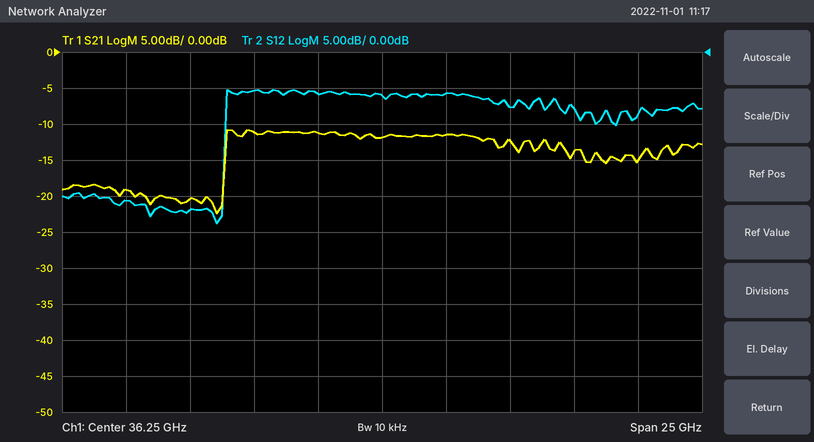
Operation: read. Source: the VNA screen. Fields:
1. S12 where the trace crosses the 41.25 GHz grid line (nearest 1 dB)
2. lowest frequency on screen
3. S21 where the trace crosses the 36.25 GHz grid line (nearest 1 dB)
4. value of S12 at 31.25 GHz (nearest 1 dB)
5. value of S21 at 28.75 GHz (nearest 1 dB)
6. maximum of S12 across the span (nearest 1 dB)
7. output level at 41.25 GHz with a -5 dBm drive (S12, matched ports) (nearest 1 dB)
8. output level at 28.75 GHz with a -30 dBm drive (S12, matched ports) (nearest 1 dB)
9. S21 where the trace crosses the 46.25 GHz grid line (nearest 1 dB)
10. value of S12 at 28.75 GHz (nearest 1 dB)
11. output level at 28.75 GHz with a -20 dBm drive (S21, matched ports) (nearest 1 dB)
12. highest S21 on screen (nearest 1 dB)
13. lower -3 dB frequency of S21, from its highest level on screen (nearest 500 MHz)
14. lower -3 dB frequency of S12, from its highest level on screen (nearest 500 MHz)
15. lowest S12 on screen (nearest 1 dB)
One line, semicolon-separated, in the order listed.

-8 dB; 23.75 GHz; -12 dB; -5 dB; -20 dB; -5 dB; -13 dBm; -52 dBm; -15 dB; -22 dB; -40 dBm; -11 dB; 30.0 GHz; 30.0 GHz; -24 dB
